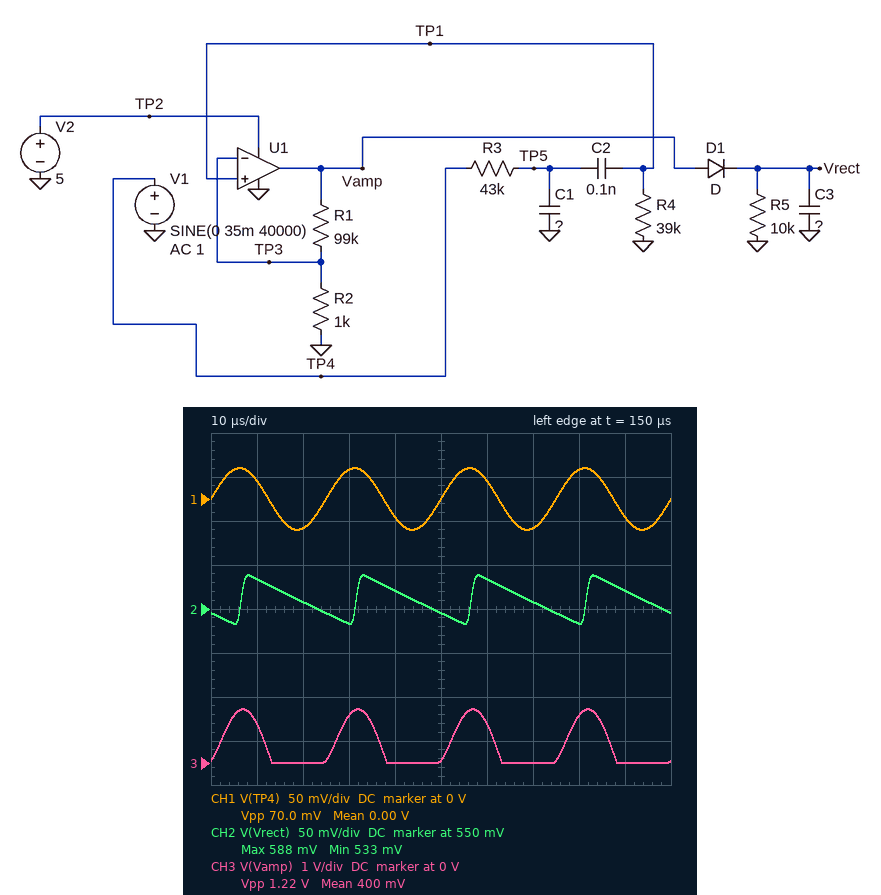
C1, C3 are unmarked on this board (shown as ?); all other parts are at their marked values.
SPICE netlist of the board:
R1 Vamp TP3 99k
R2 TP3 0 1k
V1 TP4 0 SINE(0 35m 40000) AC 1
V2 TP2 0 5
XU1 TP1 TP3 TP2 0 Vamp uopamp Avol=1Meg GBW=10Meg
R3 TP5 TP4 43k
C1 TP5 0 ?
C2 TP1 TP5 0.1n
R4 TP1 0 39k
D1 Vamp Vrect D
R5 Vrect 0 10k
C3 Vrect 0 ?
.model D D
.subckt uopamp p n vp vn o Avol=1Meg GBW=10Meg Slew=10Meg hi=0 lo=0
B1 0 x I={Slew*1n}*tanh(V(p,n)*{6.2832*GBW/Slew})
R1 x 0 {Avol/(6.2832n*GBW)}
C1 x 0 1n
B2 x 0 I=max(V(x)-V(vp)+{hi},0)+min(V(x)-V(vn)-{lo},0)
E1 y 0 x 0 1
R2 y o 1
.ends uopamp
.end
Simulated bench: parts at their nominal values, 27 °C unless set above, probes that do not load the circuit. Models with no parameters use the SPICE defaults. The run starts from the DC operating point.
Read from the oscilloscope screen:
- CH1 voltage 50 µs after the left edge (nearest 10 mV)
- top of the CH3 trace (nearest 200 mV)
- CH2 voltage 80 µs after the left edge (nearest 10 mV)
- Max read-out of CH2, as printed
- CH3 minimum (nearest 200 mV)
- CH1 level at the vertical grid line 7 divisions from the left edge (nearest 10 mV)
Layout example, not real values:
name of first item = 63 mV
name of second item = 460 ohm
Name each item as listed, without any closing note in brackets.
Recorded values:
CH1 voltage 50 µs after the left edge = 0 V
top of the CH3 trace = 1.2 V
CH2 voltage 80 µs after the left edge = 530 mV
Max read-out of CH2, as printed = 588 mV
CH3 minimum = 0 V
CH1 level at the vertical grid line 7 divisions from the left edge = -30 mV
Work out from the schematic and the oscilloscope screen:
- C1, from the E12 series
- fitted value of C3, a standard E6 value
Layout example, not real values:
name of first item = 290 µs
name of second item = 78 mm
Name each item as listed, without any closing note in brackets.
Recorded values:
C1, from the E12 series = 47 pF
fitted value of C3, a standard E6 value = 22 nF
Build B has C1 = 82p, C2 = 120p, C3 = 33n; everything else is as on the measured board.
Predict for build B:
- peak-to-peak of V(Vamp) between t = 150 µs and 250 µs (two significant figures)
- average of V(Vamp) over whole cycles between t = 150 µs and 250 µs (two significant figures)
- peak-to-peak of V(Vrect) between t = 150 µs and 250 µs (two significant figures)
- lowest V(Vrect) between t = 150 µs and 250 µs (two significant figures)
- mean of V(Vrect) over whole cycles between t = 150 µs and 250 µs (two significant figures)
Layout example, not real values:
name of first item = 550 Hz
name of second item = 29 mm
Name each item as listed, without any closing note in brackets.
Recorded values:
peak-to-peak of V(Vamp) between t = 150 µs and 250 µs = 1.1 V
average of V(Vamp) over whole cycles between t = 150 µs and 250 µs = 380 mV
peak-to-peak of V(Vrect) between t = 150 µs and 250 µs = 32 mV
lowest V(Vrect) between t = 150 µs and 250 µs = 470 mV
mean of V(Vrect) over whole cycles between t = 150 µs and 250 µs = 490 mV
